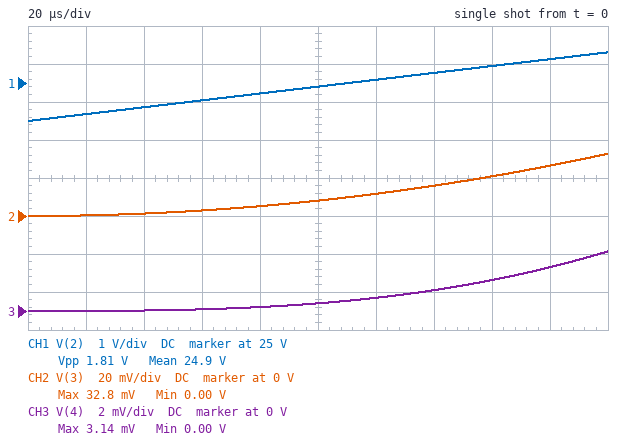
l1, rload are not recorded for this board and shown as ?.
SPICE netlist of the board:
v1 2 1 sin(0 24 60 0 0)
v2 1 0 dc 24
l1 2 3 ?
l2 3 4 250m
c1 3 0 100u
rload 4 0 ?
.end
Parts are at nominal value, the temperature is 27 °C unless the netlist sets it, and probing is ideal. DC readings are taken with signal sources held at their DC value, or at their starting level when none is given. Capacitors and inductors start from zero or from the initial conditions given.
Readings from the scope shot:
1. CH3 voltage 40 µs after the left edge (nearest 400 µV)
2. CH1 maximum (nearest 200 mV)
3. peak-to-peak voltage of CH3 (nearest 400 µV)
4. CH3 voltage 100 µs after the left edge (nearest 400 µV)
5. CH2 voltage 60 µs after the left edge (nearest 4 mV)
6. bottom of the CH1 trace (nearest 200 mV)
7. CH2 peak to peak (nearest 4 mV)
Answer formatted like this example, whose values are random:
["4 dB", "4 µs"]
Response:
["0 V", "25.8 V", "3.2 mV", "400 µV", "4 mV", "24.0 V", "32 mV"]
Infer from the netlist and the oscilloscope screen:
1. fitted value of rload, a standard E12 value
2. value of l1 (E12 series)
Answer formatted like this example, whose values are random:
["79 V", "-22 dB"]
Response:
["390 Ω", "150 mH"]
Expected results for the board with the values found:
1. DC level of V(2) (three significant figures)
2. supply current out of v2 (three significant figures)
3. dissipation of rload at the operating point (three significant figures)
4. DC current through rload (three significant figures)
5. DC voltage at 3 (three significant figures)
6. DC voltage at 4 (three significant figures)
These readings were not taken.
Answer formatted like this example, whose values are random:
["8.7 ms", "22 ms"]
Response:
["24.0 V", "61.5 mA", "1.48 W", "61.5 mA", "24.0 V", "24.0 V"]
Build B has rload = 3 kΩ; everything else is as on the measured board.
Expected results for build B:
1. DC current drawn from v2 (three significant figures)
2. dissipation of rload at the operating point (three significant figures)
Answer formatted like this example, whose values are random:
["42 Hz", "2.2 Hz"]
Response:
["8.00 mA", "192 mW"]
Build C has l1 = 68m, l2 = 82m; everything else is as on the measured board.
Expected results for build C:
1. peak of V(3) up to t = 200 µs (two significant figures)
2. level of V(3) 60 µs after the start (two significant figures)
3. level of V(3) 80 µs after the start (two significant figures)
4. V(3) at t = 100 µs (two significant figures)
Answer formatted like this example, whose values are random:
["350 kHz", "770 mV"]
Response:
["72 mV", "6.4 mV", "11 mV", "18 mV"]
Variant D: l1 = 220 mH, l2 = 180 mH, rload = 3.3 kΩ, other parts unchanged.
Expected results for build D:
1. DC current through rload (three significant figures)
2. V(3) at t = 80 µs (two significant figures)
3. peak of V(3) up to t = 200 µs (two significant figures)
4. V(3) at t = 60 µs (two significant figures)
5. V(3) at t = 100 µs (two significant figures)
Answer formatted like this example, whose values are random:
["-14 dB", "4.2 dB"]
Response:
["7.27 mA", "3.5 mV", "22 mV", "2.0 mV", "5.5 mV"]
